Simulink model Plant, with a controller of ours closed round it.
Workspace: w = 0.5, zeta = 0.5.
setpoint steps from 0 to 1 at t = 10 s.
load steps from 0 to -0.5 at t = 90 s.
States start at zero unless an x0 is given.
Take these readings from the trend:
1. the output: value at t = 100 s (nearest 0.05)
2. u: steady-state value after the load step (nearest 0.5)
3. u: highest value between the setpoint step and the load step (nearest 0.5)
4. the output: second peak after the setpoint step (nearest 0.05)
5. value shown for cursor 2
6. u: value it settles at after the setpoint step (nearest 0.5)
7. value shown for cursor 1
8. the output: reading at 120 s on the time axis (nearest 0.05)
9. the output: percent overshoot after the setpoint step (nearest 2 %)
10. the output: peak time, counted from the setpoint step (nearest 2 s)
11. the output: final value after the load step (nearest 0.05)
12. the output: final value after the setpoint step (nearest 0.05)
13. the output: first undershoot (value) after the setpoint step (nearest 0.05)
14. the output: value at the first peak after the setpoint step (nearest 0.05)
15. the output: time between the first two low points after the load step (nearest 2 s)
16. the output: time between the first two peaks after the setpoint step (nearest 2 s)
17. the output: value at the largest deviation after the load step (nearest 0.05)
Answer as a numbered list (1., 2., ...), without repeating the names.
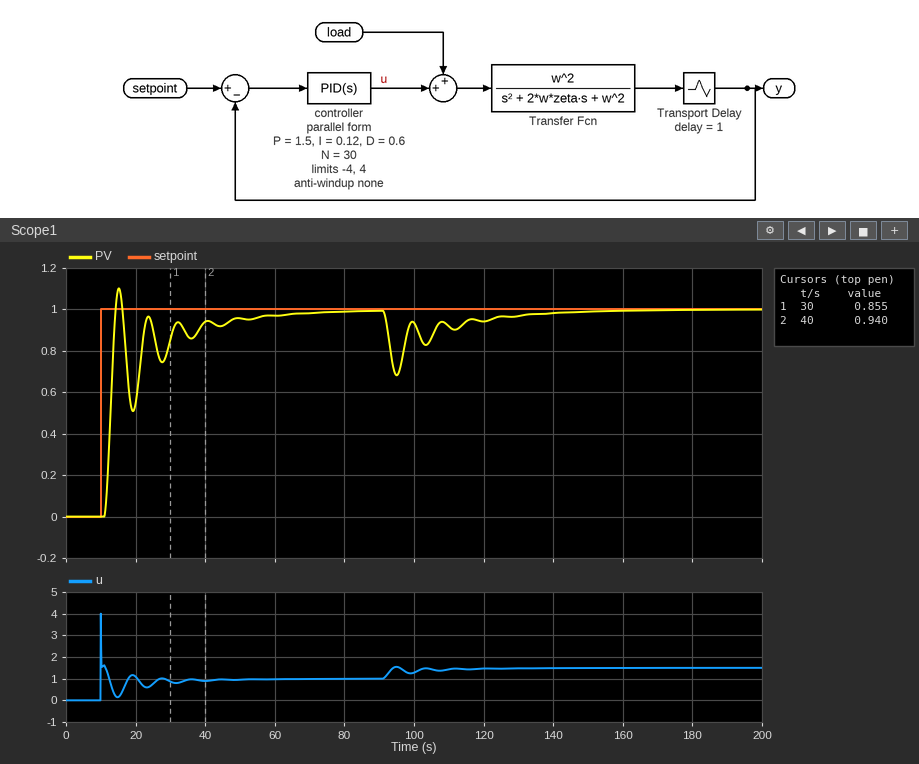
1. 0.95
2. 1.5
3. 4.0
4. 0.95
5. 0.940
6. 1.0
7. 0.855
8. 0.95
9. 10 %
10. 6 s
11. 1.00
12. 1.00
13. 0.50
14. 1.10
15. 8 s
16. 8 s
17. 0.70
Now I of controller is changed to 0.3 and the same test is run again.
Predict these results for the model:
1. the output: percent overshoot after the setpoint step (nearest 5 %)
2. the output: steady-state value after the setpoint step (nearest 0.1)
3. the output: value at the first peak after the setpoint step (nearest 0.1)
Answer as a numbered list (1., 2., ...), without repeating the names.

1. 35 %
2. 1.0
3. 1.3
